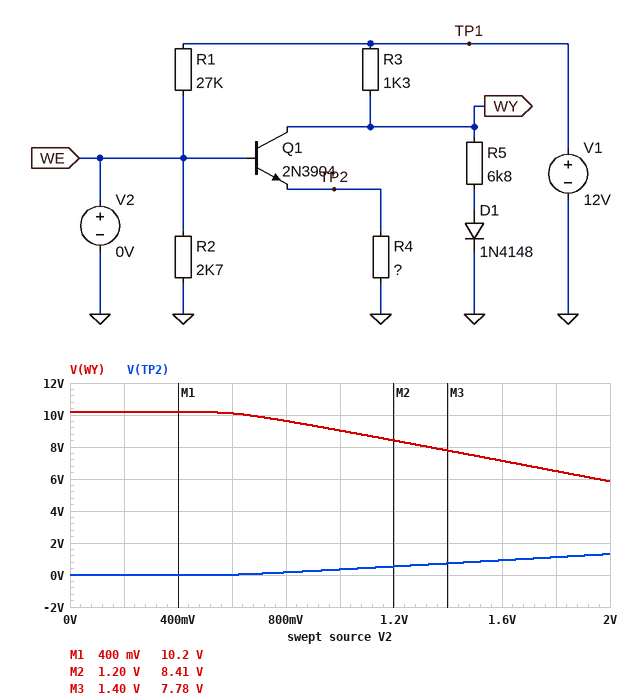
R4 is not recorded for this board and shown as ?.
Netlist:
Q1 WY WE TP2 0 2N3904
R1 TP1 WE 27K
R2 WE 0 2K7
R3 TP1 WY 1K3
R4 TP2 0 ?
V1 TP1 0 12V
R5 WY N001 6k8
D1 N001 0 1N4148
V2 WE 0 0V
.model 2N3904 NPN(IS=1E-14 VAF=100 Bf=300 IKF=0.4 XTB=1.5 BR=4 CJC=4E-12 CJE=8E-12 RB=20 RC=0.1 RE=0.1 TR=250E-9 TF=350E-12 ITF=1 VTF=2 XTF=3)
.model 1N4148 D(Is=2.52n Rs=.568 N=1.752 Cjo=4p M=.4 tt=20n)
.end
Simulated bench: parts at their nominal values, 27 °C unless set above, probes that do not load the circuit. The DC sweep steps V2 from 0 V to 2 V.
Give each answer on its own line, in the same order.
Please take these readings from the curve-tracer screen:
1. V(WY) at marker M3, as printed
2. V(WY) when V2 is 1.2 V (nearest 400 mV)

7.78 V
8.4 V
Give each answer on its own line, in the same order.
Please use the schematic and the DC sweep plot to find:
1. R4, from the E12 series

330 Ω
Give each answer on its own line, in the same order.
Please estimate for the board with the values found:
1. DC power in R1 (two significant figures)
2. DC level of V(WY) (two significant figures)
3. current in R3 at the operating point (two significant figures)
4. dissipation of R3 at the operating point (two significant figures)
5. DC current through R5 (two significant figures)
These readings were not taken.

5.3 mW
10 V
1.4 mA
2.6 mW
1.4 mA
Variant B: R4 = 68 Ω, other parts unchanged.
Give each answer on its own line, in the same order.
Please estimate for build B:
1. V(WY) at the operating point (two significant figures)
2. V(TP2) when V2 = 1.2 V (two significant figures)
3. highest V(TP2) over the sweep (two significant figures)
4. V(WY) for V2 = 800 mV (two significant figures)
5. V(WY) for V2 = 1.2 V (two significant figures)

10 V
490 mV
1.1 V
8.1 V
2.3 V
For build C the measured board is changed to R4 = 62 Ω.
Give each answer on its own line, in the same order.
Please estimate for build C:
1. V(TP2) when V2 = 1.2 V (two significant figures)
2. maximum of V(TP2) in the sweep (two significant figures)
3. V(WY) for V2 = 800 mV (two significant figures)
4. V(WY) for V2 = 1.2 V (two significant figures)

490 mV
1.1 V
7.9 V
1.6 V
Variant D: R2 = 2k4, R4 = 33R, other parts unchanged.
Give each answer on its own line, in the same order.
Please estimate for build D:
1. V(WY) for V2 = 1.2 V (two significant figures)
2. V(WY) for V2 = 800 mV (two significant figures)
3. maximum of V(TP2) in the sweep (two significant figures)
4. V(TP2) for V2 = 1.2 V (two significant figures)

420 mV
6.4 V
870 mV
400 mV
